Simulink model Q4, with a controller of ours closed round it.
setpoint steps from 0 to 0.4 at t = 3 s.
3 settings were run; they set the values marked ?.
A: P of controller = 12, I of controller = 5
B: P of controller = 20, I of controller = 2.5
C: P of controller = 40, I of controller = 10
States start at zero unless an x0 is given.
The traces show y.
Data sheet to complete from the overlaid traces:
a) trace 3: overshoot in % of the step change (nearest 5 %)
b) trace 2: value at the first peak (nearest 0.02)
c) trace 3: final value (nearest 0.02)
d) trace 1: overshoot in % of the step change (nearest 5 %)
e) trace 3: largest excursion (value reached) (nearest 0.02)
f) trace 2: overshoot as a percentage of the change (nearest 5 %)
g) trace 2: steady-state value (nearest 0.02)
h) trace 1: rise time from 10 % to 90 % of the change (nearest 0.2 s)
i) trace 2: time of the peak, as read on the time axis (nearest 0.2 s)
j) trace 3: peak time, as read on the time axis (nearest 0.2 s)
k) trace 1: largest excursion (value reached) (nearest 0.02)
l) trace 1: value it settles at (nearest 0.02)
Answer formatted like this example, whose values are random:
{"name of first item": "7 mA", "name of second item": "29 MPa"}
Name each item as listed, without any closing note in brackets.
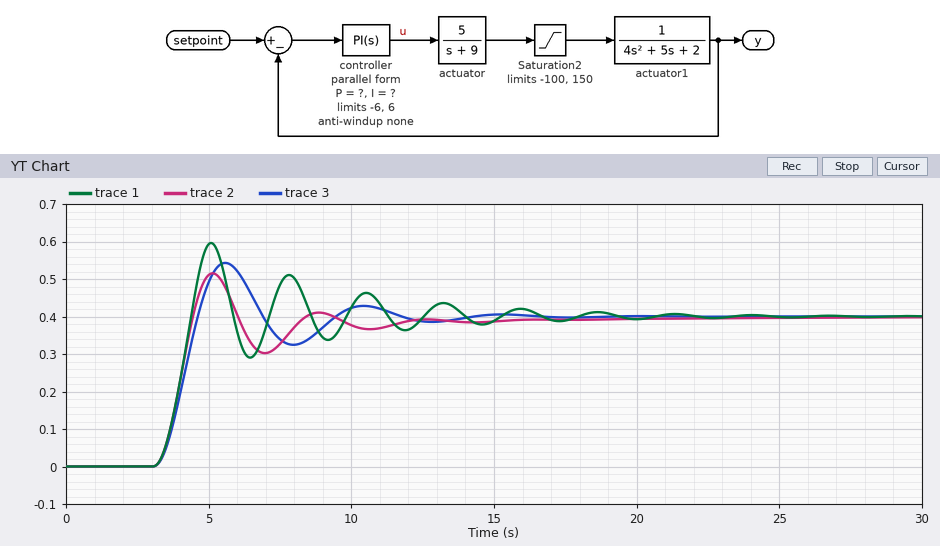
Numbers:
{"trace 3: overshoot in % of the step change": "35 %", "trace 2: value at the first peak": "0.52", "trace 3: final value": "0.40", "trace 1: overshoot in % of the step change": "50 %", "trace 3: largest excursion (value reached)": "0.54", "trace 2: overshoot as a percentage of the change": "30 %", "trace 2: steady-state value": "0.40", "trace 1: rise time from 10 % to 90 % of the change": "0.8 s", "trace 2: time of the peak, as read on the time axis": "5.2 s", "trace 3: peak time, as read on the time axis": "5.6 s", "trace 1: largest excursion (value reached)": "0.60", "trace 1: value it settles at": "0.40"}
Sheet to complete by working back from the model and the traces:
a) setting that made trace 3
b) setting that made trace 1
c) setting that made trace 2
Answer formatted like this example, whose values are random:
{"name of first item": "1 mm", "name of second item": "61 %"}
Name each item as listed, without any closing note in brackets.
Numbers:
{"setting that made trace 3": "A", "setting that made trace 1": "C", "setting that made trace 2": "B"}
